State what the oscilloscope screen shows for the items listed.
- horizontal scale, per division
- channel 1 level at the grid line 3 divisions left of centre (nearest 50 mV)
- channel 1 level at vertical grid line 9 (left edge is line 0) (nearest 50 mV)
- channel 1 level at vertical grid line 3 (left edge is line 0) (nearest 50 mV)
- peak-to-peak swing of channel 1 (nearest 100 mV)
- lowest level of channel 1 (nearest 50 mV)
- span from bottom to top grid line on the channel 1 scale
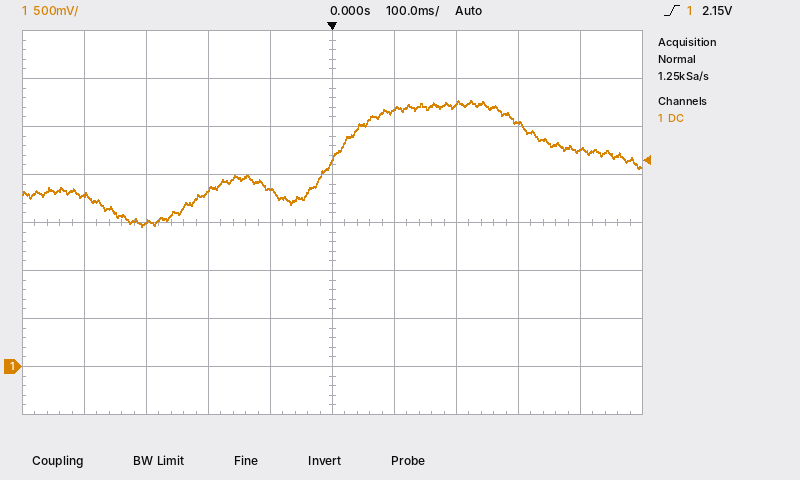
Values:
100 ms
1.50 V
2.25 V
1.85 V
1.30 V
1.45 V
4 V
